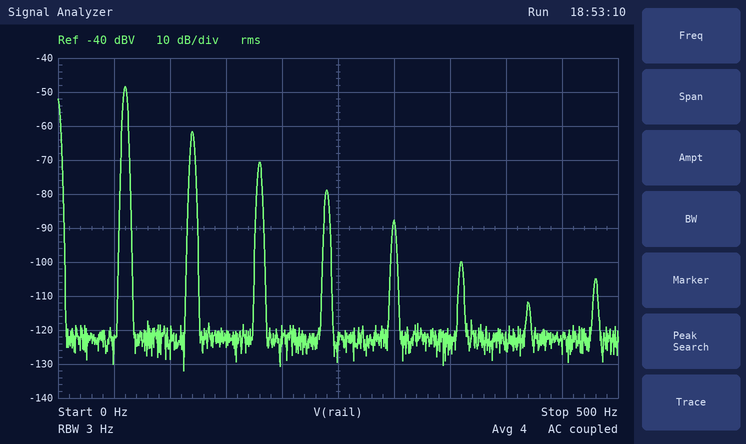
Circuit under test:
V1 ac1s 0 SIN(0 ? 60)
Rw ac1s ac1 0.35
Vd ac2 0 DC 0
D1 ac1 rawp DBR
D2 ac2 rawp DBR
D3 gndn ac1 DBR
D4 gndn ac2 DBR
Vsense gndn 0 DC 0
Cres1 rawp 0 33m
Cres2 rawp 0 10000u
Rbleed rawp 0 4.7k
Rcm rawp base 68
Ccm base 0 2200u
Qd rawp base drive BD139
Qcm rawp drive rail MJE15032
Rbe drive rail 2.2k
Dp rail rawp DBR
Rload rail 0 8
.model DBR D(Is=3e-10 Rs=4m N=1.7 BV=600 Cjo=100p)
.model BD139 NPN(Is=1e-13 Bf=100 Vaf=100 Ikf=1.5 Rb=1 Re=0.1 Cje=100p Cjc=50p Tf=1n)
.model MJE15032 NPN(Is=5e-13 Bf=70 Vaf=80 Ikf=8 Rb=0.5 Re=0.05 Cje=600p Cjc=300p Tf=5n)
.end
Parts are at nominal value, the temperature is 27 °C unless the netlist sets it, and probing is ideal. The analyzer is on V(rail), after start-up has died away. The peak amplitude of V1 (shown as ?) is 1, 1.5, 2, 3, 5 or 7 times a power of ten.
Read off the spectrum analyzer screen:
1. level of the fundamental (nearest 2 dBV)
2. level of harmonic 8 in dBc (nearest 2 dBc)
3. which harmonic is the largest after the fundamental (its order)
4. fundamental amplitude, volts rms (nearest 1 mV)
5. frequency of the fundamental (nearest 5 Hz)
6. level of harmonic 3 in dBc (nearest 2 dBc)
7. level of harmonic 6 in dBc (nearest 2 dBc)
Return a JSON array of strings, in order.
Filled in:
["-48 dBV", "-56 dBc", "2", "4 mV", "60 Hz", "-22 dBc", "-52 dBc"]
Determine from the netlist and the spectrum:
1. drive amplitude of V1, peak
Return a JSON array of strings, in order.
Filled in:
["30 V"]
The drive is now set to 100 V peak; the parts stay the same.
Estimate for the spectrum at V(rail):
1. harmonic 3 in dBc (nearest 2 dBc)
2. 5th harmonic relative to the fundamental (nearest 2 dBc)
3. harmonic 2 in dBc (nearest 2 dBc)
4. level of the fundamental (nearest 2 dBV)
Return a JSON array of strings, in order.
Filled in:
["-10 dBc", "-12 dBc", "-6 dBc", "-32 dBV"]
